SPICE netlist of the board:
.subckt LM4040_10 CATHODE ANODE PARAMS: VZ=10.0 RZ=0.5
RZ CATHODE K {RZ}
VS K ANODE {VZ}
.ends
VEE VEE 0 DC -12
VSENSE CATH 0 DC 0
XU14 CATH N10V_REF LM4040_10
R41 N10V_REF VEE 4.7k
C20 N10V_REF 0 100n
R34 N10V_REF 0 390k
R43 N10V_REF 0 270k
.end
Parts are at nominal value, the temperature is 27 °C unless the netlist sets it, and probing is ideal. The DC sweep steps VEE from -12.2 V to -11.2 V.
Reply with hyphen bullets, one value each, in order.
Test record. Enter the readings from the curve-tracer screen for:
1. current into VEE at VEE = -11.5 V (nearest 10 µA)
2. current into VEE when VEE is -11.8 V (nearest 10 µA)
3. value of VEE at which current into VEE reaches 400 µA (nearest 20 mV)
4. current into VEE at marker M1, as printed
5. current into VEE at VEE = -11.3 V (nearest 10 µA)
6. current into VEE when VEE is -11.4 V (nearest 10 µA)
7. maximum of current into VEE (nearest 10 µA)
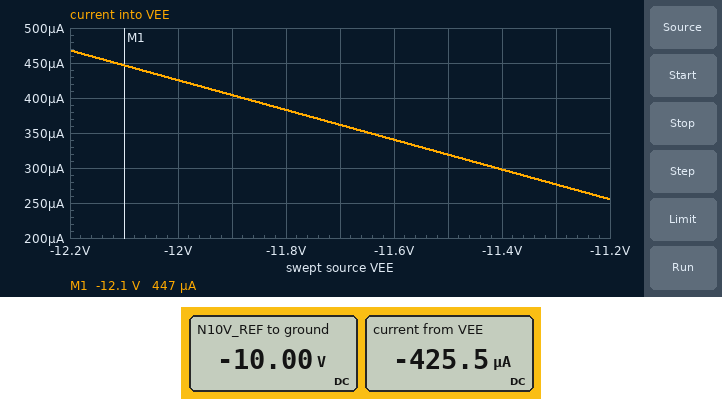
- 320 µA
- 380 µA
- -11.88 V
- 447 µA
- 280 µA
- 300 µA
- 470 µA
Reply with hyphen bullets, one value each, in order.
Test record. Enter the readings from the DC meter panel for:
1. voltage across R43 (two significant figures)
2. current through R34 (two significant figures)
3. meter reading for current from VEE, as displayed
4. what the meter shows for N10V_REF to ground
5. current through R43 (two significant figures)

- 10 V
- 26 µA
- -425.5 µA
- -10.00 V
- 37 µA
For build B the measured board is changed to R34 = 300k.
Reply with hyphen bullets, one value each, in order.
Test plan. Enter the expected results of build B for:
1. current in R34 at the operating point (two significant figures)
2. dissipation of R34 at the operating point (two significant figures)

- 33 µA
- 330 µW
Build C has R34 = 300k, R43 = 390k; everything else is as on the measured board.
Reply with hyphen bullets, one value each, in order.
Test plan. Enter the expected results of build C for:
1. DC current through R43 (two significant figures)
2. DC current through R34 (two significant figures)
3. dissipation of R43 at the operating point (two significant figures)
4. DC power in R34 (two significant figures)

- 26 µA
- 33 µA
- 260 µW
- 330 µW
